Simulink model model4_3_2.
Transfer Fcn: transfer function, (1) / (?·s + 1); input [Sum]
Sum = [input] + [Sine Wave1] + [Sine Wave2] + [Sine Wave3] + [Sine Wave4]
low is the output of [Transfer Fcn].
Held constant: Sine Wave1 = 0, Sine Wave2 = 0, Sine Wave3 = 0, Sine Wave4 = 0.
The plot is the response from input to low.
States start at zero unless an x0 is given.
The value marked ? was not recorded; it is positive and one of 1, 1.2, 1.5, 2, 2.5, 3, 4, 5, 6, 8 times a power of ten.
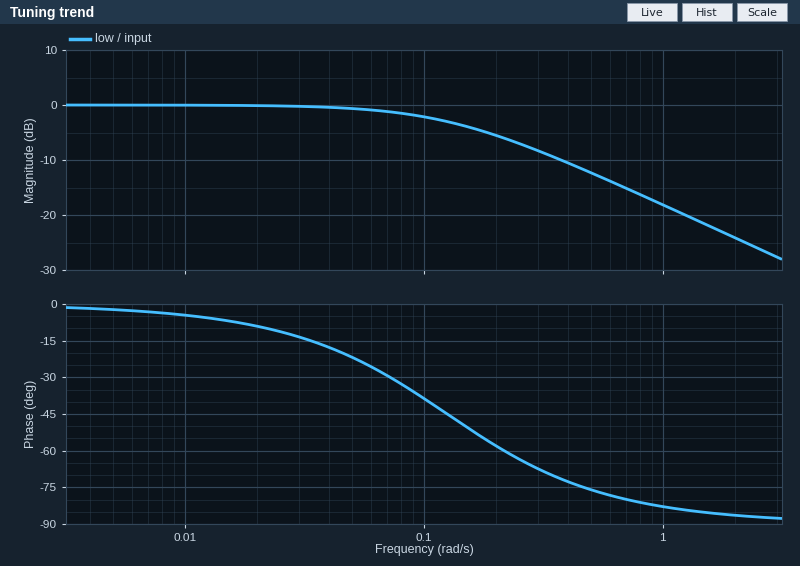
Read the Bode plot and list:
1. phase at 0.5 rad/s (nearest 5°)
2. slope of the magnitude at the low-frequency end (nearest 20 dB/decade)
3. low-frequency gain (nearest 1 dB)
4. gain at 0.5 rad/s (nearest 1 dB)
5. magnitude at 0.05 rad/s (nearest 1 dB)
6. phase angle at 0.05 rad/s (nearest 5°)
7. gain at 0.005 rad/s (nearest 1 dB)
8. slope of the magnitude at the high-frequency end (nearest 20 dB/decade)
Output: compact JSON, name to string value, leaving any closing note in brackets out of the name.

{"phase at 0.5 rad/s": "-75°", "slope of the magnitude at the low-frequency end": "0 dB/decade", "low-frequency gain": "0 dB", "gain at 0.5 rad/s": "-12 dB", "magnitude at 0.05 rad/s": "-1 dB", "phase angle at 0.05 rad/s": "-20°", "gain at 0.005 rad/s": "0 dB", "slope of the magnitude at the high-frequency end": "-20 dB/decade"}
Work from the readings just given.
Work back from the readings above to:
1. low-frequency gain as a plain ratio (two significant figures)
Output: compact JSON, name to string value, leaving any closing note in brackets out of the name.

{"low-frequency gain as a plain ratio": "1.0"}
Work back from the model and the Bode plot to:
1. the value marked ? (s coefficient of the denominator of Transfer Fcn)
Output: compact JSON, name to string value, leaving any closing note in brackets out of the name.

{"the value marked ?": "8"}
